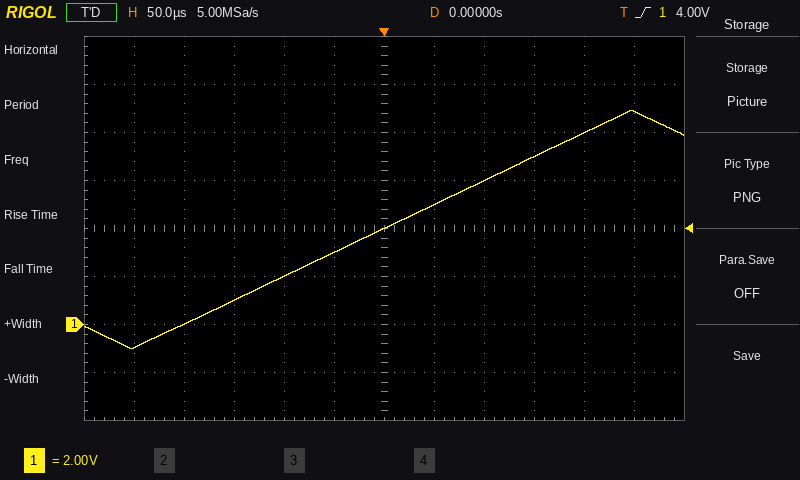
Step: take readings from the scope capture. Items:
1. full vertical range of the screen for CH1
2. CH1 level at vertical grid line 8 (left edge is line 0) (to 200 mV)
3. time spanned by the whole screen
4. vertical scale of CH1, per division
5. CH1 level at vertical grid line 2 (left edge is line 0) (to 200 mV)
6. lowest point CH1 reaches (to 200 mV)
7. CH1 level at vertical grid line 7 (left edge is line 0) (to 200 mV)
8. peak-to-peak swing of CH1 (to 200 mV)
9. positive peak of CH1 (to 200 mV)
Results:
16 V
6.0 V
600 µs
2 V
0.0 V
-1.0 V
5.0 V
10.0 V
9.0 V
